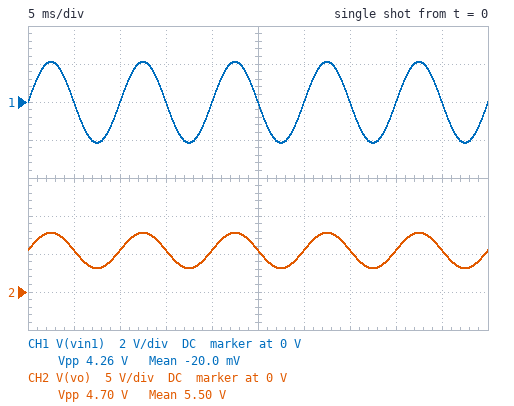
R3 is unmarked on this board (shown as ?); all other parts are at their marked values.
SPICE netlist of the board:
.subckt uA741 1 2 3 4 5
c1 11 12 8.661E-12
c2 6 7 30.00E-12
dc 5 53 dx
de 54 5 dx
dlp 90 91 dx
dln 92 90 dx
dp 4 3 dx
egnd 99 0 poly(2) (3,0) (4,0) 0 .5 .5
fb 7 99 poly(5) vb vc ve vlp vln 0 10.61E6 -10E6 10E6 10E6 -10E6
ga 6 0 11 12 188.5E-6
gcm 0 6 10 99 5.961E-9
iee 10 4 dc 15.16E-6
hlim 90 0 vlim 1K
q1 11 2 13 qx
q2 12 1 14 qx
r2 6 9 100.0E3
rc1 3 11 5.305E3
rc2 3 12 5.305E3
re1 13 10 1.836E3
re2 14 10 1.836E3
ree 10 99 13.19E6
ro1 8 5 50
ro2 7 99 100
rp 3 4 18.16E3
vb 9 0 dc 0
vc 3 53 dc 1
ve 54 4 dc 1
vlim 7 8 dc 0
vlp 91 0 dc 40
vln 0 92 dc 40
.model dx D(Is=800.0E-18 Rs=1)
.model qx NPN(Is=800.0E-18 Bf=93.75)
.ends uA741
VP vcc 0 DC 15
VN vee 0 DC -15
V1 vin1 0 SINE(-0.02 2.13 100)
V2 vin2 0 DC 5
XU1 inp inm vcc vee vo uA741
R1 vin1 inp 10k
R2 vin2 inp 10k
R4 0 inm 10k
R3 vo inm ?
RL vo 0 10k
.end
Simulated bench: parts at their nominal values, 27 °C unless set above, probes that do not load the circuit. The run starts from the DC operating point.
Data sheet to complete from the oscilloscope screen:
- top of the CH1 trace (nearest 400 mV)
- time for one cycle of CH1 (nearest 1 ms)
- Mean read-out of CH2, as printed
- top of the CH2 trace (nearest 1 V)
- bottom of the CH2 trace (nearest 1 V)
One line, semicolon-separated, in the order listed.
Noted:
2.0 V; 10 ms; 5.50 V; 8 V; 3 V
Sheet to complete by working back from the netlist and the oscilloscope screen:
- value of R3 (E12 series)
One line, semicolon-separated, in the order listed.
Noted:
12 kΩ
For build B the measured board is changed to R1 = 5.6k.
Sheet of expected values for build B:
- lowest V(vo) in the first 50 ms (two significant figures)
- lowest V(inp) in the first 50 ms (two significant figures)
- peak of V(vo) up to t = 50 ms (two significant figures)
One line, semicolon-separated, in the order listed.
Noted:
920 mV; 420 mV; 6.9 V
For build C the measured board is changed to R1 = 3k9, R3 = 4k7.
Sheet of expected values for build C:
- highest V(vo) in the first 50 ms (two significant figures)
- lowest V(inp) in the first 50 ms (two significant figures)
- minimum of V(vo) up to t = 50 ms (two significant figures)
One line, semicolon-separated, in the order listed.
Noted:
4.3 V; -140 mV; -210 mV
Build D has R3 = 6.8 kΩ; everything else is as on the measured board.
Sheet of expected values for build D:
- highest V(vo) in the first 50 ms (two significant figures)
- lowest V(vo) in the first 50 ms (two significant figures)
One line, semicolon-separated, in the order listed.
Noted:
6.0 V; 2.4 V
